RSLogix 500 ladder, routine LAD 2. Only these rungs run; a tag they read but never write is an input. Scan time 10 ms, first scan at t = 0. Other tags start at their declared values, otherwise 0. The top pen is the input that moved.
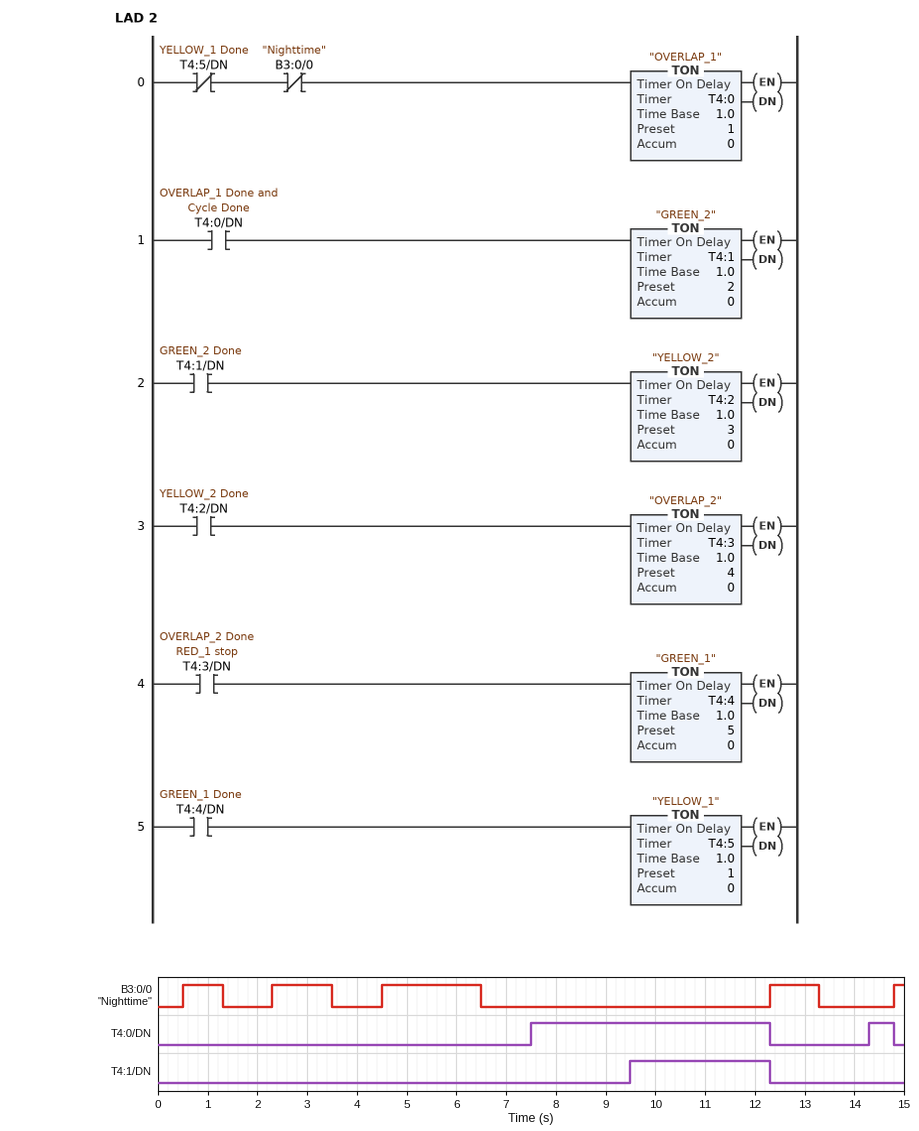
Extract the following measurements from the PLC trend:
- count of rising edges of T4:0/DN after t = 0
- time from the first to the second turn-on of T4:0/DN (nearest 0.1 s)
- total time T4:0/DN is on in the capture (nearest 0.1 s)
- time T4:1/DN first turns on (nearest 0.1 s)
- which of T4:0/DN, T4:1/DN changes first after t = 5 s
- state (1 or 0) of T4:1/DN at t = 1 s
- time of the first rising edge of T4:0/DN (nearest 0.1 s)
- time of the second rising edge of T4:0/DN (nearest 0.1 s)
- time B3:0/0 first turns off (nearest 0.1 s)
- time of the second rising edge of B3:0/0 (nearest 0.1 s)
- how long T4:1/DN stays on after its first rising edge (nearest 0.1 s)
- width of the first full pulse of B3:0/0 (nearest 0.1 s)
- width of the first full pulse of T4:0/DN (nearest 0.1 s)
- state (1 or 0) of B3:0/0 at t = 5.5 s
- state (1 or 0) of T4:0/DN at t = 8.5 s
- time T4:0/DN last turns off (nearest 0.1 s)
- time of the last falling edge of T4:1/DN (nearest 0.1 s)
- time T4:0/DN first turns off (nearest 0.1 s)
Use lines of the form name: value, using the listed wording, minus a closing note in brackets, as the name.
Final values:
count of rising edges of T4:0/DN after t = 0: 2
time from the first to the second turn-on of T4:0/DN: 6.8 s
total time T4:0/DN is on in the capture: 5.3 s
time T4:1/DN first turns on: 9.5 s
which of T4:0/DN, T4:1/DN changes first after t = 5 s: T4:0/DN
state (1 or 0) of T4:1/DN at t = 1 s: 0
time of the first rising edge of T4:0/DN: 7.5 s
time of the second rising edge of T4:0/DN: 14.3 s
time B3:0/0 first turns off: 1.3 s
time of the second rising edge of B3:0/0: 2.3 s
how long T4:1/DN stays on after its first rising edge: 2.8 s
width of the first full pulse of B3:0/0: 0.8 s
width of the first full pulse of T4:0/DN: 4.8 s
state (1 or 0) of B3:0/0 at t = 5.5 s: 1
state (1 or 0) of T4:0/DN at t = 8.5 s: 1
time T4:0/DN last turns off: 14.8 s
time of the last falling edge of T4:1/DN: 12.3 s
time T4:0/DN first turns off: 12.3 s
